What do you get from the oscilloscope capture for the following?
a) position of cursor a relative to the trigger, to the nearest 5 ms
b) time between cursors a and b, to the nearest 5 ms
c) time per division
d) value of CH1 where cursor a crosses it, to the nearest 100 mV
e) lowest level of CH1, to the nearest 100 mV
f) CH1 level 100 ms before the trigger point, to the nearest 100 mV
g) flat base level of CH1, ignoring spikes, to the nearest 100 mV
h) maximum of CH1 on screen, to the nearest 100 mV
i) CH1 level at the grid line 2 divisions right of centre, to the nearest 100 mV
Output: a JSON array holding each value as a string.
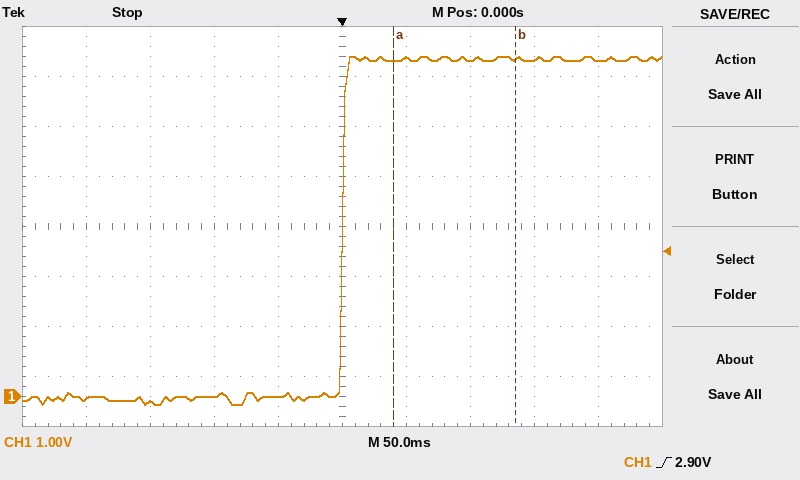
["+40 ms", "95 ms", "50 ms", "6.7 V", "-200 mV", "0.0 V", "0.0 V", "6.8 V", "6.7 V"]
